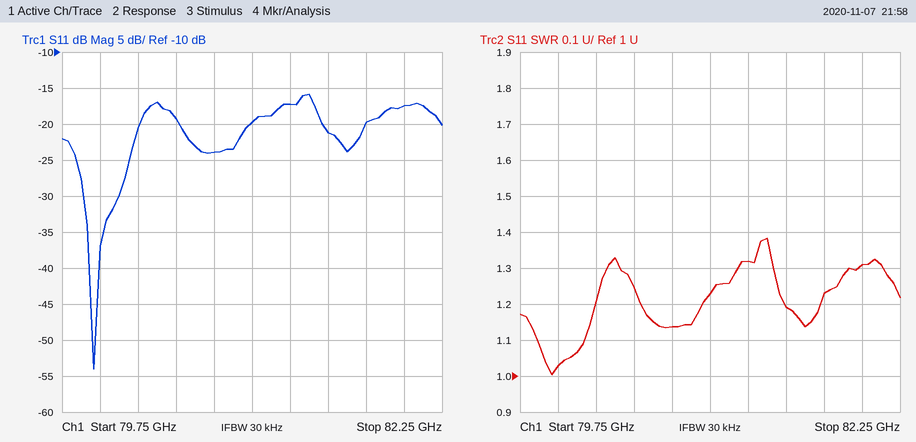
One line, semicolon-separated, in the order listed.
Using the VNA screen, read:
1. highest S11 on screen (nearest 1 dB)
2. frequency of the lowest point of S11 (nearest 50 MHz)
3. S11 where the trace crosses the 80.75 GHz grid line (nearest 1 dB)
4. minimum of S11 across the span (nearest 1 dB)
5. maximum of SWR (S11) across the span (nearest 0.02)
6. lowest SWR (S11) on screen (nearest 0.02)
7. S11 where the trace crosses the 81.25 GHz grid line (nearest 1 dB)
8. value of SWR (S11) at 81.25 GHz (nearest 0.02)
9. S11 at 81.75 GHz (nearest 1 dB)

-16 dB; 79.95 GHz; -24 dB; -54 dB; 1.38; 1.00; -17 dB; 1.32; -20 dB
